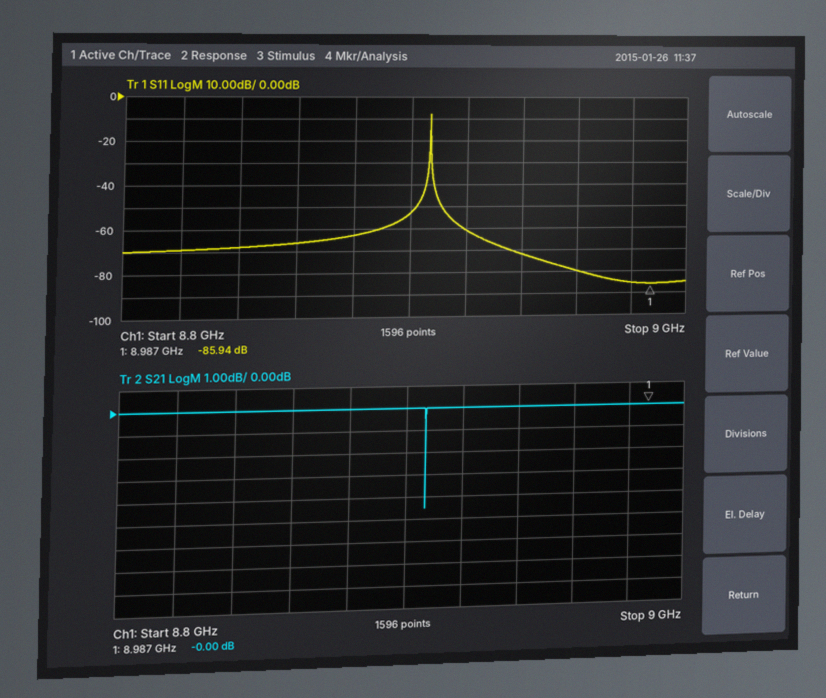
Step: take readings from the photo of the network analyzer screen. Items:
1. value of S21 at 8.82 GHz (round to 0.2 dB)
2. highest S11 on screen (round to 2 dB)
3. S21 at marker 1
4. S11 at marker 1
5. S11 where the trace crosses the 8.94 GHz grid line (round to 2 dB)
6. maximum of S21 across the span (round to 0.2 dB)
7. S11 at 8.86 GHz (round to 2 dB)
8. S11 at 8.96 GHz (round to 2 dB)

0.0 dB
-8 dB
-0.00 dB
-85.94 dB
-72 dB
0.0 dB
-66 dB
-80 dB
